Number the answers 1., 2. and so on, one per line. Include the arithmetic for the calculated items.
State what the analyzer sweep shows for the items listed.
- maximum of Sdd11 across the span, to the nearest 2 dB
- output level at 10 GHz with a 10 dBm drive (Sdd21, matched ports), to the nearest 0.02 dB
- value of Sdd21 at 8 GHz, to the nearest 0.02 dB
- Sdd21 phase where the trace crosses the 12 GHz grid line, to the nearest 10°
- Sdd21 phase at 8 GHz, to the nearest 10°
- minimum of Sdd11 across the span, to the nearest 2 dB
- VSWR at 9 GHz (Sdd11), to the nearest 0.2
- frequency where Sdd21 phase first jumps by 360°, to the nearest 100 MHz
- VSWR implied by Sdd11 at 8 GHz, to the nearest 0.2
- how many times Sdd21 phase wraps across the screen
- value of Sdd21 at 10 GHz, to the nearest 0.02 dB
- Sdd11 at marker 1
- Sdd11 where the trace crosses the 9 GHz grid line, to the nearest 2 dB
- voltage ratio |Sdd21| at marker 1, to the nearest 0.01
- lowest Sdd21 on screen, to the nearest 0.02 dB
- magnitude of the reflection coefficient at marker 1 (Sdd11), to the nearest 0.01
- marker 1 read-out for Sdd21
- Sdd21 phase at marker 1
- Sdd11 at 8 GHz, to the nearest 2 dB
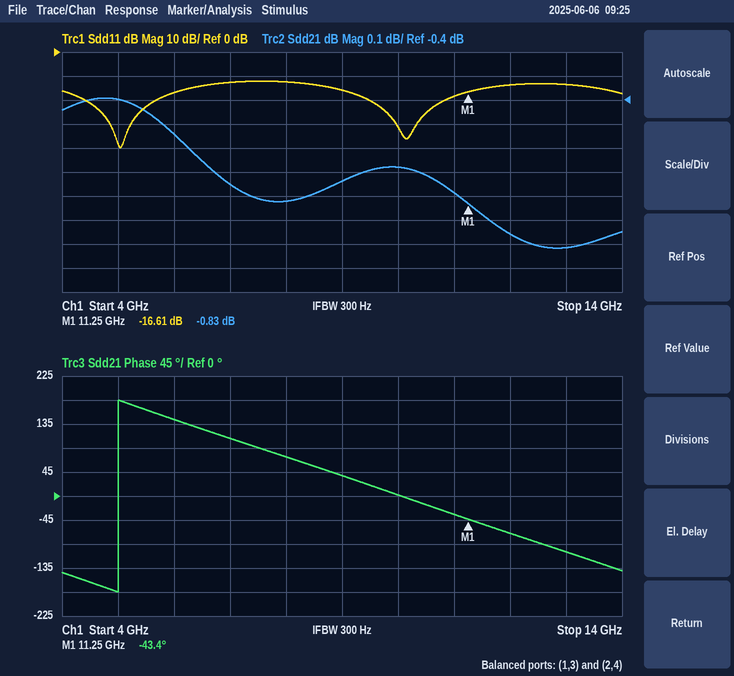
1. -12 dB
2. 10 dBm + (-0.68 dB) = 9.32 dBm
3. -0.82 dB
4. -70°
5. 70°
6. -40 dB
7. |Γ| = 10^(-16/20) = 0.1585; VSWR = (1 + 0.1585)/(1 − 0.1585) ≈ 1.4
8. 5.0 GHz
9. |Γ| = 10^(-12/20) = 0.2512; VSWR = (1 + 0.2512)/(1 − 0.2512) ≈ 1.67, so 1.6 to the nearest 0.2
10. 1
11. -0.68 dB
12. -16.61 dB
13. -16 dB
14. 10^(-0.83/20) ≈ 0.91
15. -1.02 dB
16. 10^(-16.61/20) ≈ 0.15
17. -0.83 dB
18. -43.4°
19. -12 dB
